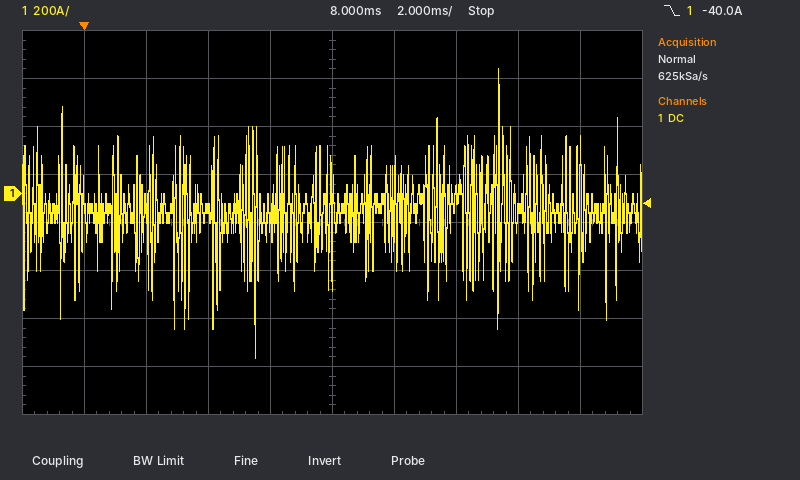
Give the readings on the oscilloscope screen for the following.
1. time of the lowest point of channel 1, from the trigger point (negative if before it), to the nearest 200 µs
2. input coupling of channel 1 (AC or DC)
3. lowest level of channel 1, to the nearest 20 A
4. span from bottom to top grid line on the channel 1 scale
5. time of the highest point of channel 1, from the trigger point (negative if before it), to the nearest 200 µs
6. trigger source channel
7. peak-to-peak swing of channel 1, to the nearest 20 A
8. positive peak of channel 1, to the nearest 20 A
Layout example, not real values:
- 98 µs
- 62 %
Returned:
- +5.6 ms
- DC
- -680 A
- 1.6 kA
- +13.4 ms
- channel 1
- 1.20 kA
- 520 A
